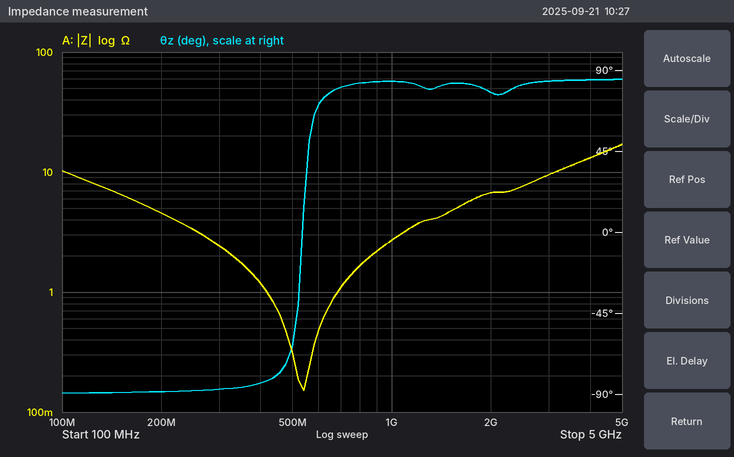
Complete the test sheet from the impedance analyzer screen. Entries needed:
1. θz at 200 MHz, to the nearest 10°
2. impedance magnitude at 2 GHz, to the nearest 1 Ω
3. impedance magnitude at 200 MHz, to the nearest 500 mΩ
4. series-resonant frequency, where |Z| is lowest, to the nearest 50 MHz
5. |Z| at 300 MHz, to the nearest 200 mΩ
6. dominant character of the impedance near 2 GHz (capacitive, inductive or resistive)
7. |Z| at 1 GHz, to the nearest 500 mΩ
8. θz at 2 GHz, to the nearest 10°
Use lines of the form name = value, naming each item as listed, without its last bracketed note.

θz at 200 MHz, to the nearest 10° = -90°
impedance magnitude at 2 GHz, to the nearest 1 Ω = 7 Ω
impedance magnitude at 200 MHz, to the nearest 500 mΩ = 4.5 Ω
series-resonant frequency, where |Z| is lowest, to the nearest 50 MHz = 550 MHz
|Z| at 300 MHz, to the nearest 200 mΩ = 2.4 Ω
dominant character of the impedance near 2 GHz = inductive
|Z| at 1 GHz, to the nearest 500 mΩ = 2.5 Ω
θz at 2 GHz, to the nearest 10° = 80°
